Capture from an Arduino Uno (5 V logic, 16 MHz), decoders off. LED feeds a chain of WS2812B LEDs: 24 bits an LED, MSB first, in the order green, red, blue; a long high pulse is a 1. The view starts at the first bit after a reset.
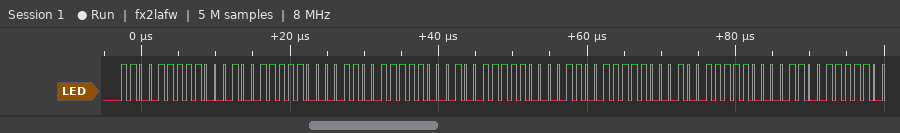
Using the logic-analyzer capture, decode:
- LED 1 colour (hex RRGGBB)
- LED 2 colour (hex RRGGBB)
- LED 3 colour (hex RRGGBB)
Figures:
#89CFF0
#89CFF0
#89CFF0
